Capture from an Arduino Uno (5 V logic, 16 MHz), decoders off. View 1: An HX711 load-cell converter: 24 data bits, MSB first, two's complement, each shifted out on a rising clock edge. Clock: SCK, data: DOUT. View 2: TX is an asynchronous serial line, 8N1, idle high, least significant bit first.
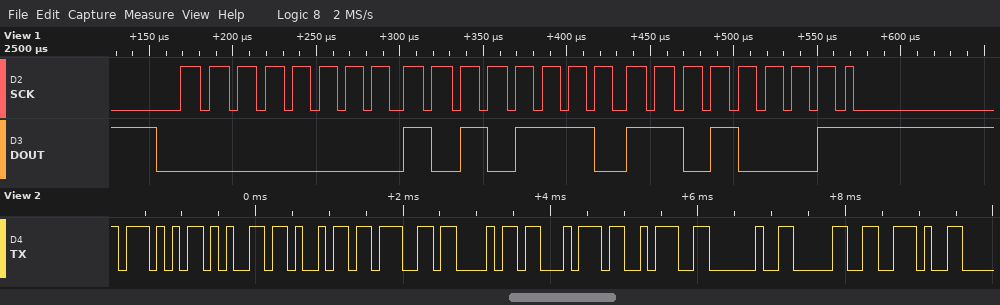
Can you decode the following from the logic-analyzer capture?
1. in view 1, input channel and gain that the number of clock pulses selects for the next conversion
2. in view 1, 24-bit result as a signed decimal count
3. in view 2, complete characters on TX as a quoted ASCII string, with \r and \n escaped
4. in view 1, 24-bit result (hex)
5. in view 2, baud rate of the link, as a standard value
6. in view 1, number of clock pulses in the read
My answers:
channel A, gain 128
44753
"Weight: 0."
0x00AED1
9600 baud
25
